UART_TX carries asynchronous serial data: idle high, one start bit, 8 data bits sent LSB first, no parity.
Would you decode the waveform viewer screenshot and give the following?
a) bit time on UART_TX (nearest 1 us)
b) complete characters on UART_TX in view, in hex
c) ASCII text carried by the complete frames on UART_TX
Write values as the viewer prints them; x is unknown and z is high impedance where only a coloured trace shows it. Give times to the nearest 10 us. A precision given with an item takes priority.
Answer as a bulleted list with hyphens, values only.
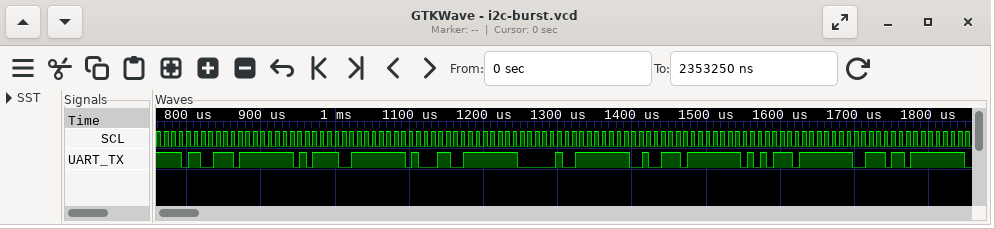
- 9 us
- 73, 3D, 31, 20, 72, 75, 6E
- "s=1 run"
